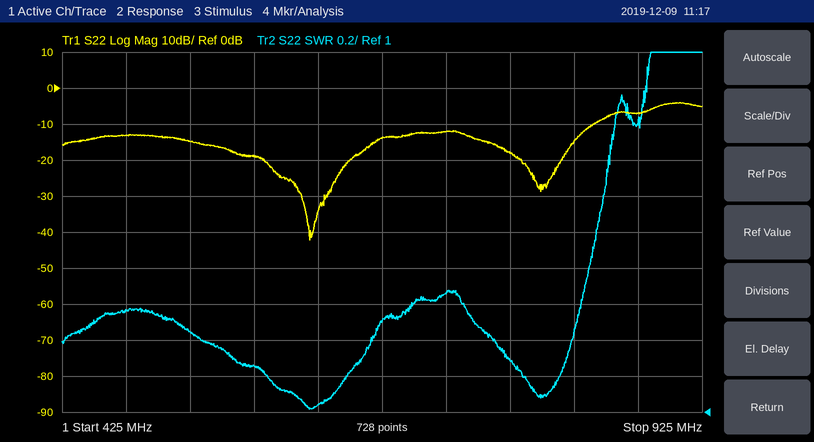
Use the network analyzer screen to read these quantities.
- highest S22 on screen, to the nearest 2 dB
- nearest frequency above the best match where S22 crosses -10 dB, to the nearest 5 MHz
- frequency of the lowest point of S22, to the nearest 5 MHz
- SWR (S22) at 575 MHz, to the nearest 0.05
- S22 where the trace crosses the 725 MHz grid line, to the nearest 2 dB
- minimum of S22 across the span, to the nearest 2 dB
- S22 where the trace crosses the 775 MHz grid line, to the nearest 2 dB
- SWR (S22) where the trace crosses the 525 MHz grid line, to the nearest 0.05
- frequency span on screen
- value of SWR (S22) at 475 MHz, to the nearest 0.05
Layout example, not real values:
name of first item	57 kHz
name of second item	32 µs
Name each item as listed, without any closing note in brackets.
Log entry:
highest S22 on screen, to the nearest 2 dB	-4 dB
nearest frequency above the best match where S22 crosses -10 dB, to the nearest 5 MHz	840 MHz
frequency of the lowest point of S22, to the nearest 5 MHz	620 MHz
SWR (S22) at 575 MHz, to the nearest 0.05	1.25
S22 where the trace crosses the 725 MHz grid line, to the nearest 2 dB	-12 dB
minimum of S22 across the span, to the nearest 2 dB	-42 dB
S22 where the trace crosses the 775 MHz grid line, to the nearest 2 dB	-18 dB
SWR (S22) where the trace crosses the 525 MHz grid line, to the nearest 0.05	1.45
frequency span on screen	500 MHz
value of SWR (S22) at 475 MHz, to the nearest 0.05	1.55
